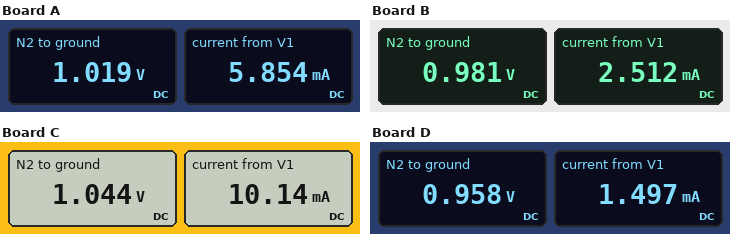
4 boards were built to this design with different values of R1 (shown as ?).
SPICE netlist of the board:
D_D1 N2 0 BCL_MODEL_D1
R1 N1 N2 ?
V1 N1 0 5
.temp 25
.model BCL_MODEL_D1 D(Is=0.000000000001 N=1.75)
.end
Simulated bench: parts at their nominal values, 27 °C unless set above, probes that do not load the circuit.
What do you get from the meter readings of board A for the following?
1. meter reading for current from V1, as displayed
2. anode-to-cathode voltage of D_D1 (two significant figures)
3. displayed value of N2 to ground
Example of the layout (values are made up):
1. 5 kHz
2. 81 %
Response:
1. 5.854 mA
2. 1.0 V
3. 1.019 V
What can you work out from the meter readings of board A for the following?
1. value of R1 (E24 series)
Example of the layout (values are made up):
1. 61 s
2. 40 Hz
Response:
1. 680 Ω
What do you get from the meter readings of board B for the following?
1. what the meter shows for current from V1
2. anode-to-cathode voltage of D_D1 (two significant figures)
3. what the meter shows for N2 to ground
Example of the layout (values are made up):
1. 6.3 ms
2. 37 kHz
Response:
1. 2.512 mA
2. 980 mV
3. 0.981 V
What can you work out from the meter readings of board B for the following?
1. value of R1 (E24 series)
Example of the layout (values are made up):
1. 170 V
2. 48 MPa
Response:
1. 1.6 kΩ
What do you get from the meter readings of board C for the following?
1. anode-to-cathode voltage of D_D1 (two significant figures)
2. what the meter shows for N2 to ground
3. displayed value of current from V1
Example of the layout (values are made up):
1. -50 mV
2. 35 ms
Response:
1. 1.0 V
2. 1.044 V
3. 10.14 mA
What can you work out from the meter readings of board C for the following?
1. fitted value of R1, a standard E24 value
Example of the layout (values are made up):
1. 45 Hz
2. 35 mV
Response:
1. 390 Ω
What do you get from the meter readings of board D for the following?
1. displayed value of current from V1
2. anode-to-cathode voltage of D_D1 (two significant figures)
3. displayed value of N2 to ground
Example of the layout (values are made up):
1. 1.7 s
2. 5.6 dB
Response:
1. 1.497 mA
2. 960 mV
3. 0.958 V
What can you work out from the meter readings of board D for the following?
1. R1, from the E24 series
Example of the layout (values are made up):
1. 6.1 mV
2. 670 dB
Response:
1. 2.7 kΩ
